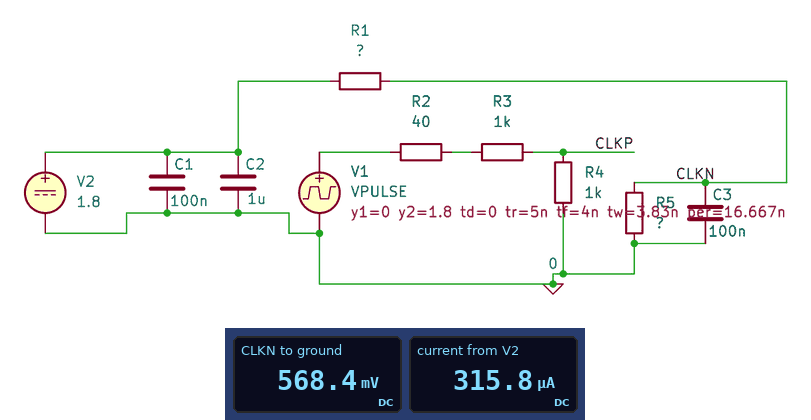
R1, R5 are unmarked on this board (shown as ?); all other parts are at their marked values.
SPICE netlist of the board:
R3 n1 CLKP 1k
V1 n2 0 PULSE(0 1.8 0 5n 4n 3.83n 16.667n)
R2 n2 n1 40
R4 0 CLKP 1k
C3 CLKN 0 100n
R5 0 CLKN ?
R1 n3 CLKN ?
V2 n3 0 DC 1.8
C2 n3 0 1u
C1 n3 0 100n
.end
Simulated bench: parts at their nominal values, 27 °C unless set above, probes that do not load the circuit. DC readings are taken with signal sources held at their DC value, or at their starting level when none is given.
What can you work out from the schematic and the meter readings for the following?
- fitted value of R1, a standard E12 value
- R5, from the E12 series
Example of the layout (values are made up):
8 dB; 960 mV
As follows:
3.9 kΩ; 1.8 kΩ
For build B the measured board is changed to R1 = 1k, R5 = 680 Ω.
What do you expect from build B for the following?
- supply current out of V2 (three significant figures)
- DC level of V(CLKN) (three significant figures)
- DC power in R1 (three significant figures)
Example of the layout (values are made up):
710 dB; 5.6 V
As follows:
1.07 mA; 729 mV; 1.15 mW
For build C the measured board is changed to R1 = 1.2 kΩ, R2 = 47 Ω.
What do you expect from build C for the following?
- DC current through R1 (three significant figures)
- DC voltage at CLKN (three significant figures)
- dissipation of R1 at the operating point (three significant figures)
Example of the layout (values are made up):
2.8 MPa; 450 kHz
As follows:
600 µA; 1.08 V; 432 µW
